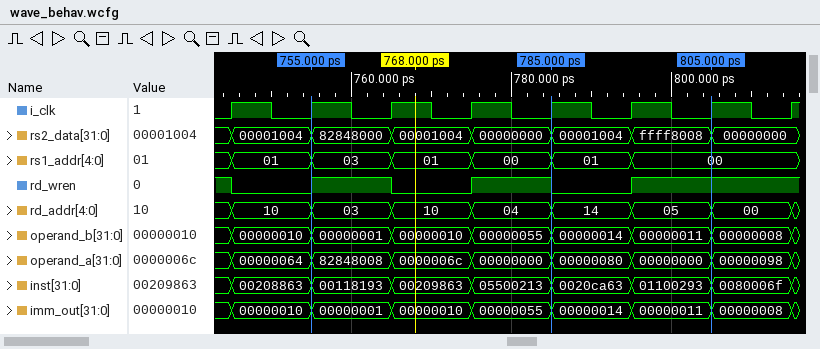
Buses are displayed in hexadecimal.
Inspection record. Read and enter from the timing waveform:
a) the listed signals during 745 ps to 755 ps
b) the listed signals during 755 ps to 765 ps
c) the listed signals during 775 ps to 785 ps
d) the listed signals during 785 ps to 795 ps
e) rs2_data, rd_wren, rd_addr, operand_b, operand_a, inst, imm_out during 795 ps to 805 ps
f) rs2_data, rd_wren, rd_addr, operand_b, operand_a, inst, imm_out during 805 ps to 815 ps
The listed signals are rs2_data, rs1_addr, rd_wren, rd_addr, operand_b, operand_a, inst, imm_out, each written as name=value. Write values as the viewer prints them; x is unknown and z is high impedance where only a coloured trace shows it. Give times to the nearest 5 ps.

rs2_data=00001004, rs1_addr=01, rd_wren=0, rd_addr=10, operand_b=00000010, operand_a=00000064, inst=00208863, imm_out=00000010
rs2_data=82848000, rs1_addr=03, rd_wren=1, rd_addr=03, operand_b=00000001, operand_a=82848008, inst=00118193, imm_out=00000001
rs2_data=00000000, rs1_addr=00, rd_wren=1, rd_addr=04, operand_b=00000055, operand_a=00000000, inst=05500213, imm_out=00000055
rs2_data=00001004, rs1_addr=01, rd_wren=0, rd_addr=14, operand_b=00000014, operand_a=00000080, inst=0020ca63, imm_out=00000014
rs2_data=ffff8008, rd_wren=1, rd_addr=05, operand_b=00000011, operand_a=00000000, inst=01100293, imm_out=00000011
rs2_data=00000000, rd_wren=1, rd_addr=00, operand_b=00000008, operand_a=00000098, inst=0080006f, imm_out=00000008
